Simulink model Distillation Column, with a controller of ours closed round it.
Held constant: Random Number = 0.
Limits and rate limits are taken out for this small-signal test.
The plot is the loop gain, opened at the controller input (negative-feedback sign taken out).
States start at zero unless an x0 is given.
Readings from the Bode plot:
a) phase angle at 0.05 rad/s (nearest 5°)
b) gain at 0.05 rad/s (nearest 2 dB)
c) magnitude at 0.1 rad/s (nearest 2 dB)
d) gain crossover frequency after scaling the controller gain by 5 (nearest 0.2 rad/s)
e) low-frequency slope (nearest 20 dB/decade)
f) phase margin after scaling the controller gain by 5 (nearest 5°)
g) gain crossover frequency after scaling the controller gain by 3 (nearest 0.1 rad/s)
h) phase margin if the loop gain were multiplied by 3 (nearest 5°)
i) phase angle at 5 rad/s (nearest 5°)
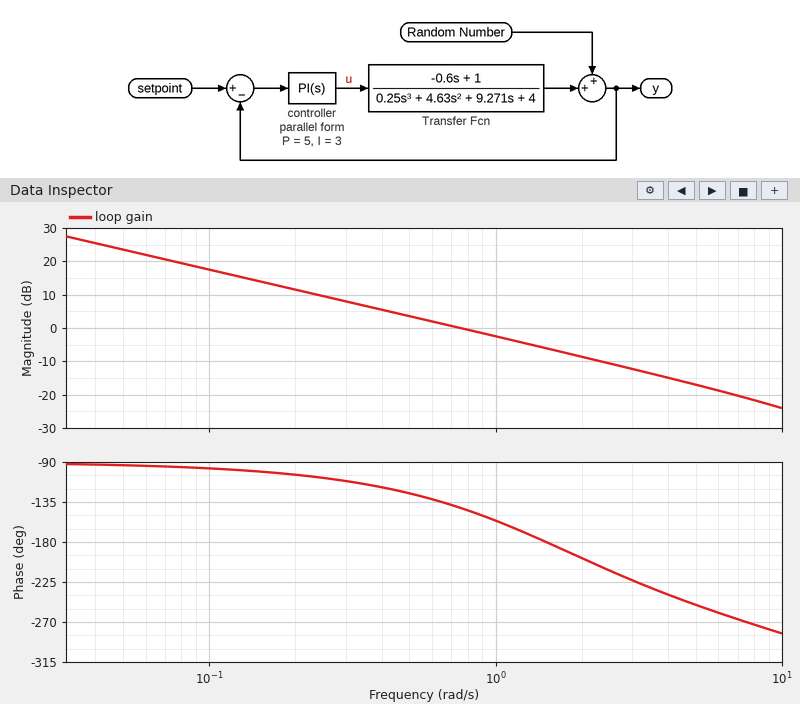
-95°
24 dB
18 dB
3.6 rad/s
-20 dB/decade
-55°
2.2 rad/s
-25°
-250°
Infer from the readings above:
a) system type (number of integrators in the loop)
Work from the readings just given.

1
